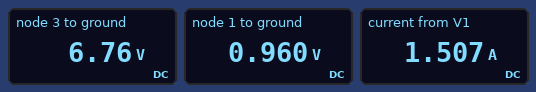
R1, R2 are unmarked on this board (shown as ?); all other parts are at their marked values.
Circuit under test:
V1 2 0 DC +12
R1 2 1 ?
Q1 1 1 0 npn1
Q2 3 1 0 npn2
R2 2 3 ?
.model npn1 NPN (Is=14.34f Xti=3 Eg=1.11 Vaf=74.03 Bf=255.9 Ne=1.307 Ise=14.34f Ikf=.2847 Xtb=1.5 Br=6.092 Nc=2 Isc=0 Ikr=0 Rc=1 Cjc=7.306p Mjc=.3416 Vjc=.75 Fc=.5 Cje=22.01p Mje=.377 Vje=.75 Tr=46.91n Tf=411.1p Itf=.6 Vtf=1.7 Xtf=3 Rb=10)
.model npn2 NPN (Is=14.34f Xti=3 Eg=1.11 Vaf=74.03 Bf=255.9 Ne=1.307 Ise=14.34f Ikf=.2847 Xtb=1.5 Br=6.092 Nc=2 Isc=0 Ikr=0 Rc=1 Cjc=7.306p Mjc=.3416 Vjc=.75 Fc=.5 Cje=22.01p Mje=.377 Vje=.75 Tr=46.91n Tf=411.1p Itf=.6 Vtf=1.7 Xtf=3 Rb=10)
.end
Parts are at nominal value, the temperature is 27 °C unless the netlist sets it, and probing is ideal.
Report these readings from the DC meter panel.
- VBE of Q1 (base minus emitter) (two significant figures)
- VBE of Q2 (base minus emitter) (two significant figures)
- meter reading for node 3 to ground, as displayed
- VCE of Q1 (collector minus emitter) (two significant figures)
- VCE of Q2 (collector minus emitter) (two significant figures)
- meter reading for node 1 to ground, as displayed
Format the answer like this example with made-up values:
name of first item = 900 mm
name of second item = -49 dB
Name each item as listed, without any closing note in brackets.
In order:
VBE of Q1 (base minus emitter) = 960 mV
VBE of Q2 (base minus emitter) = 960 mV
meter reading for node 3 to ground, as displayed = 6.76 V
VCE of Q1 (collector minus emitter) = 960 mV
VCE of Q2 (collector minus emitter) = 6.8 V
meter reading for node 1 to ground, as displayed = 0.960 V
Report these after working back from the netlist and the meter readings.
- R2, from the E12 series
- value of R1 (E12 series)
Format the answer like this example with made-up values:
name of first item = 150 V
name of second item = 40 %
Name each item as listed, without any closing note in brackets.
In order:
R2, from the E12 series = 6.8 Ω
value of R1 = 15 Ω
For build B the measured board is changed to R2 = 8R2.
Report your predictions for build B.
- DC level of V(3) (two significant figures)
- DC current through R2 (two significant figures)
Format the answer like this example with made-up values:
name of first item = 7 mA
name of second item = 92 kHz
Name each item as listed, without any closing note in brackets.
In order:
DC level of V(3) = 5.8 V
DC current through R2 = 760 mA
